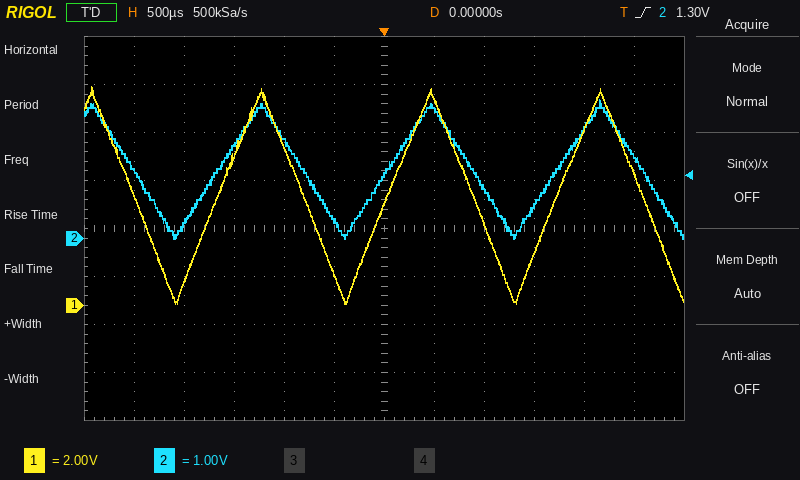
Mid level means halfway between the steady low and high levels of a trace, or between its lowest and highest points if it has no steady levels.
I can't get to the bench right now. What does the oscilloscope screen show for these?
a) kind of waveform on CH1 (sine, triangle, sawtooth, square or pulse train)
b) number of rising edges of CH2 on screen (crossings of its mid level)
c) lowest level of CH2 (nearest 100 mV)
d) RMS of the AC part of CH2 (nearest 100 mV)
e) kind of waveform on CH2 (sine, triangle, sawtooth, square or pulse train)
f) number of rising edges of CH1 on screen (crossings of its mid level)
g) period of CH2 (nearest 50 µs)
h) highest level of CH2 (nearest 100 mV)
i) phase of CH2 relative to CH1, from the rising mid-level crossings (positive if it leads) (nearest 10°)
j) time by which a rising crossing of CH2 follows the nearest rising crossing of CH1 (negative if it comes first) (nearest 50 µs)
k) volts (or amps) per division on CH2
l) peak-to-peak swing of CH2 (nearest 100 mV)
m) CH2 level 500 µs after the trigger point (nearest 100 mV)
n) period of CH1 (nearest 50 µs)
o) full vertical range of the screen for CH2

triangle
3
0.0 V
800 mV
triangle
3
1.70 ms
2.9 V
0°
0 µs
1 V
2.9 V
2.7 V
1.70 ms
8 V
